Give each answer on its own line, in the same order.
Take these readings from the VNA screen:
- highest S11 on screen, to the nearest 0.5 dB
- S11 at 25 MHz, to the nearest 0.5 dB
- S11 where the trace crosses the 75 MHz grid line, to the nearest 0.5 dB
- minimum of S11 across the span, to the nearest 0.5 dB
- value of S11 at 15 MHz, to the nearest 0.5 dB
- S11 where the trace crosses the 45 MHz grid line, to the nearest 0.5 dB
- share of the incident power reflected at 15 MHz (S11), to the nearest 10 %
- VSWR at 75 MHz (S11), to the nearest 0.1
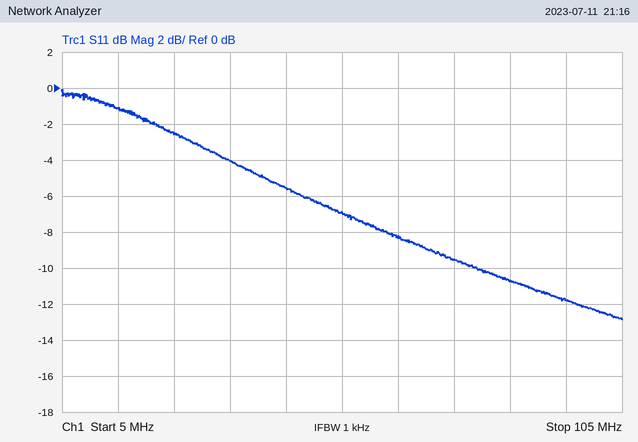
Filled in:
0.0 dB
-2.5 dB
-9.5 dB
-13.0 dB
-1.0 dB
-5.5 dB
80 %
2.0
